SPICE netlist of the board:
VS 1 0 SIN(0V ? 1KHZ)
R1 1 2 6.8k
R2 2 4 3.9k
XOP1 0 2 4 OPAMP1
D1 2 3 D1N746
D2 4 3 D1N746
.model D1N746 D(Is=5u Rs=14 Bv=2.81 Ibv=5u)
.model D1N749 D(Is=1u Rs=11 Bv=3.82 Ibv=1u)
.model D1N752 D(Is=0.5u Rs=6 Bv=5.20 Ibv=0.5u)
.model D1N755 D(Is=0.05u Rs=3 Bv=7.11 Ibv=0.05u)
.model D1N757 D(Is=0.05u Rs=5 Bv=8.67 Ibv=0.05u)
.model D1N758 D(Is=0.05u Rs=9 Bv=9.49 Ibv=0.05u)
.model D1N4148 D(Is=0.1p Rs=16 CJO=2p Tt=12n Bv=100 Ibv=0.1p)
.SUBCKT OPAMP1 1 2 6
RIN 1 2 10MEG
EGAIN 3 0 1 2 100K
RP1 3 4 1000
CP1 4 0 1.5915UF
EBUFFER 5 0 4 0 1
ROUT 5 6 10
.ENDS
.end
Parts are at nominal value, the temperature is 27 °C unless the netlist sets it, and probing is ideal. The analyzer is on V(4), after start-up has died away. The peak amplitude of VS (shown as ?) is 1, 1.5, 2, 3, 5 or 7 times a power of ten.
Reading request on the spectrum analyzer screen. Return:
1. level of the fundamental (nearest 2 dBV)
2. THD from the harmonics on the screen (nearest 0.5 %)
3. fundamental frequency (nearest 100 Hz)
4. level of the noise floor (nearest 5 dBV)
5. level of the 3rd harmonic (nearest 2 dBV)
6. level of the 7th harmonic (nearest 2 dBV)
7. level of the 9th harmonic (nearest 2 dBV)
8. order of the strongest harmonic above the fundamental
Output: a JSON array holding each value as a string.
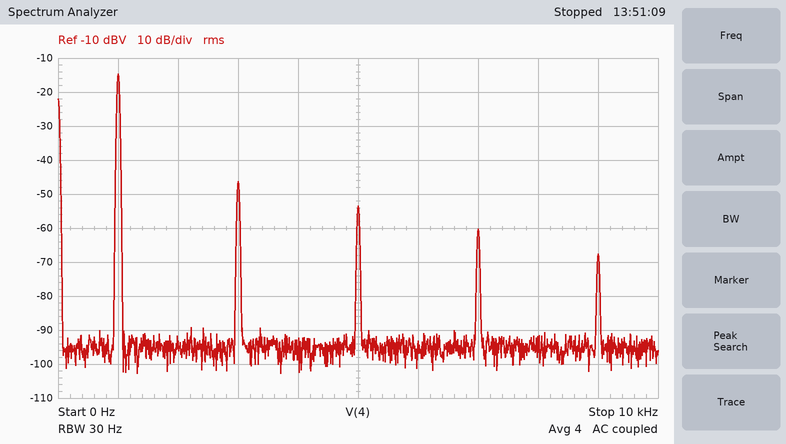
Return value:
["-14 dBV", "3.0 %", "1.0 kHz", "-95 dBV", "-46 dBV", "-60 dBV", "-68 dBV", "3"]
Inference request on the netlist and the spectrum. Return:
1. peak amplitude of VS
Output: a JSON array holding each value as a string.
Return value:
["500 mV"]
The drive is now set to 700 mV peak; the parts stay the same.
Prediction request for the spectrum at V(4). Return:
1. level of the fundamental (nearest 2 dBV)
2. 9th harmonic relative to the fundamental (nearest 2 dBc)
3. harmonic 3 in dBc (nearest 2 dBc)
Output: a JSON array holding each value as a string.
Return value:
["-12 dBV", "-50 dBc", "-34 dBc"]
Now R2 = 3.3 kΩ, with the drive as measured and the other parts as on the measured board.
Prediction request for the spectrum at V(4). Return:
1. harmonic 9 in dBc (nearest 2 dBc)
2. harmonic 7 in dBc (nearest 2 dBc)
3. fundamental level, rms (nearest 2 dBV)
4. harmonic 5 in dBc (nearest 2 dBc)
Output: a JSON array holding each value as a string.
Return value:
["-56 dBc", "-48 dBc", "-16 dBV", "-40 dBc"]
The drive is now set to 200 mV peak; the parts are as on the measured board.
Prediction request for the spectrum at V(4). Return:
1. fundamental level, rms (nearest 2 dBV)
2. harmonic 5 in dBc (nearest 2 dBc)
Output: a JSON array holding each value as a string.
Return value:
["-24 dBV", "-48 dBc"]
